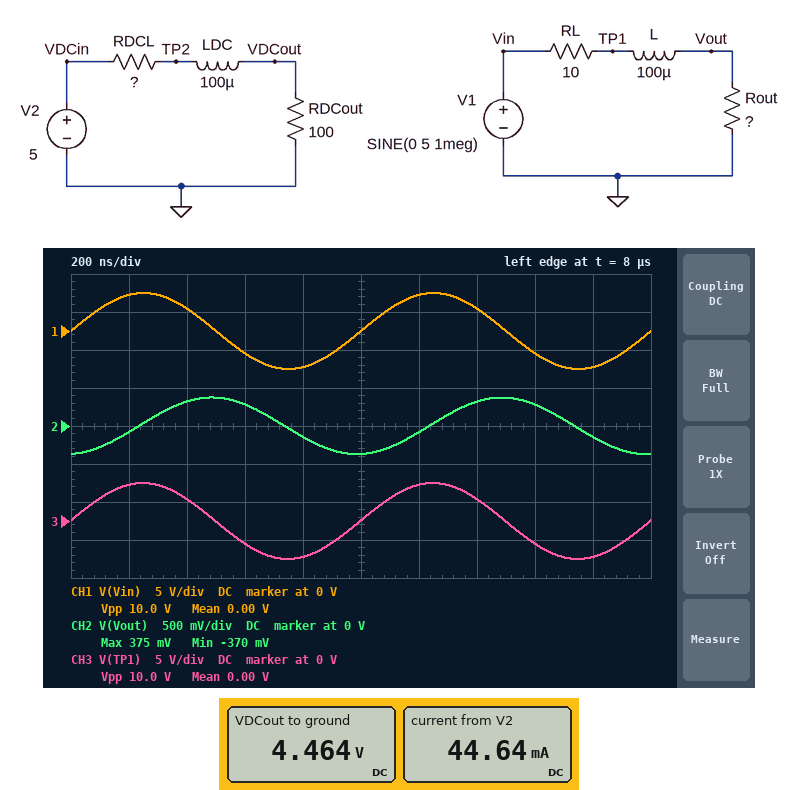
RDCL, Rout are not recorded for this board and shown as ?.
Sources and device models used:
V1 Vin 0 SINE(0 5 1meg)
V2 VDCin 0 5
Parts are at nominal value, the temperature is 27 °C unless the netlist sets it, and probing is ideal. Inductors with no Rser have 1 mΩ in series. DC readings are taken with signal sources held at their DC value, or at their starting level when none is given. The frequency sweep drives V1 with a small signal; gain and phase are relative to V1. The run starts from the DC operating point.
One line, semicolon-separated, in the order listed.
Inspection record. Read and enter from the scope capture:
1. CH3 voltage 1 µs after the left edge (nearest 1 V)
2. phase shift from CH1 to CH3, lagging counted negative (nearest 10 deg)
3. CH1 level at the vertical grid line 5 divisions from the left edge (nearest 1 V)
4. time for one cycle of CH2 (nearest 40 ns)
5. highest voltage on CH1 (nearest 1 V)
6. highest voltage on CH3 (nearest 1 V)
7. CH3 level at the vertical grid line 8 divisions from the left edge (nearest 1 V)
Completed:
0 V; 0 deg; 0 V; 1.00 µs; 5 V; 5 V; -3 V
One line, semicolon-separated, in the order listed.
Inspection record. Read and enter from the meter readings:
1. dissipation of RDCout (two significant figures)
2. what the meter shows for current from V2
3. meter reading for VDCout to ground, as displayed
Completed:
200 mW; 44.64 mA; 4.464 V
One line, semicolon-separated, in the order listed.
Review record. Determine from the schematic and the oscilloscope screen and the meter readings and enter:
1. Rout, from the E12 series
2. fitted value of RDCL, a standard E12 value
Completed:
47 Ω; 12 Ω
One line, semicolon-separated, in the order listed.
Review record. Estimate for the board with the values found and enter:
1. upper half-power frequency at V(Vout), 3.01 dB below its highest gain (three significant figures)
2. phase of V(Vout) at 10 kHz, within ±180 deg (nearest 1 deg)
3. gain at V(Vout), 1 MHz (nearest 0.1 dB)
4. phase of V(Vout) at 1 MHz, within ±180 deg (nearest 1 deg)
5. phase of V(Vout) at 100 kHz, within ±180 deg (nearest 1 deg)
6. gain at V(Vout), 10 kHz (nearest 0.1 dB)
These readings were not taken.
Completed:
90.7 kHz; -6 deg; -22.6 dB; -85 deg; -48 deg; -1.7 dB
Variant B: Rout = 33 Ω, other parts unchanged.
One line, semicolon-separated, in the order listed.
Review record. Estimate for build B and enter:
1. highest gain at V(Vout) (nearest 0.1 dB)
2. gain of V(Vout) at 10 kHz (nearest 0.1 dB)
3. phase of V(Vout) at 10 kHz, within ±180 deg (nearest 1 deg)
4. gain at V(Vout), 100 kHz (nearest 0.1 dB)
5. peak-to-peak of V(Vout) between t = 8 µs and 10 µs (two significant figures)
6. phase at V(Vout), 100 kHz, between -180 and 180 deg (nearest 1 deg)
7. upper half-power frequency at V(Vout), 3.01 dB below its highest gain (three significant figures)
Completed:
-2.3 dB; -2.4 dB; -8 deg; -7.3 dB; 530 mV; -56 deg; 68.4 kHz
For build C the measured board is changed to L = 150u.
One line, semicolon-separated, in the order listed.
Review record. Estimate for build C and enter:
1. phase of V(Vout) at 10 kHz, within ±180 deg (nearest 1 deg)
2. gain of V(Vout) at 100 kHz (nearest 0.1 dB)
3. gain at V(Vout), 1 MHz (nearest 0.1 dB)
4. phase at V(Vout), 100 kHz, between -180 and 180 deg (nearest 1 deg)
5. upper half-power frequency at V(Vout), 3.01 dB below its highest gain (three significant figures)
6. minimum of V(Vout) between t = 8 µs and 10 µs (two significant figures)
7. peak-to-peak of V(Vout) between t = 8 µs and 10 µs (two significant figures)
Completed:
-9 deg; -7.4 dB; -26.1 dB; -59 deg; 60.5 kHz; -240 mV; 500 mV
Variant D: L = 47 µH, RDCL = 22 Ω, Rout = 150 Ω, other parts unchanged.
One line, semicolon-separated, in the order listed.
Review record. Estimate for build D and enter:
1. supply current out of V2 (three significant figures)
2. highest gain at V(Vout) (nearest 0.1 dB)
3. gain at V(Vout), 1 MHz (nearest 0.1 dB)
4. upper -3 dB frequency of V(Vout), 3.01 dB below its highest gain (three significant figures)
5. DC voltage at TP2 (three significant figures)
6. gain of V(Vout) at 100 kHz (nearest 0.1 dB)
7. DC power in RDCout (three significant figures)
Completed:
41.0 mA; -0.6 dB; -7.0 dB; 542 kHz; 4.10 V; -0.7 dB; 168 mW
